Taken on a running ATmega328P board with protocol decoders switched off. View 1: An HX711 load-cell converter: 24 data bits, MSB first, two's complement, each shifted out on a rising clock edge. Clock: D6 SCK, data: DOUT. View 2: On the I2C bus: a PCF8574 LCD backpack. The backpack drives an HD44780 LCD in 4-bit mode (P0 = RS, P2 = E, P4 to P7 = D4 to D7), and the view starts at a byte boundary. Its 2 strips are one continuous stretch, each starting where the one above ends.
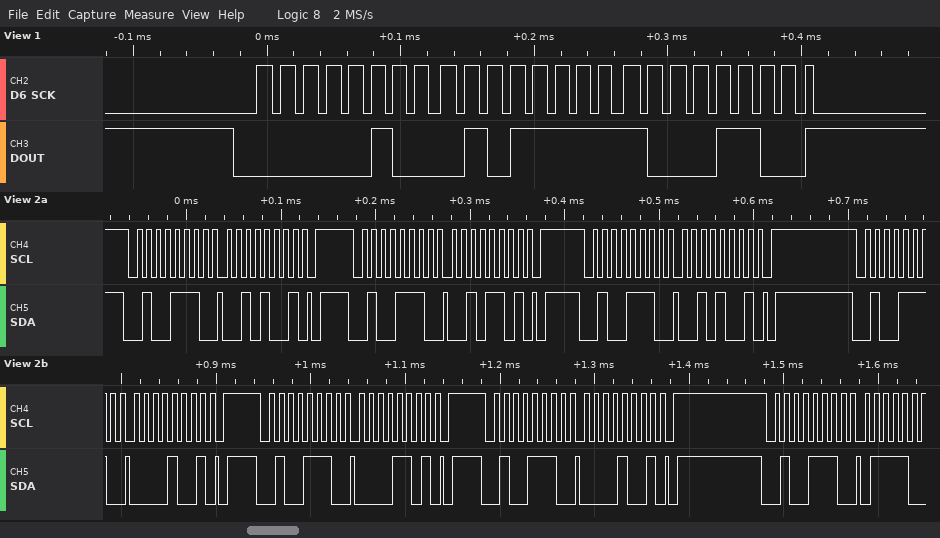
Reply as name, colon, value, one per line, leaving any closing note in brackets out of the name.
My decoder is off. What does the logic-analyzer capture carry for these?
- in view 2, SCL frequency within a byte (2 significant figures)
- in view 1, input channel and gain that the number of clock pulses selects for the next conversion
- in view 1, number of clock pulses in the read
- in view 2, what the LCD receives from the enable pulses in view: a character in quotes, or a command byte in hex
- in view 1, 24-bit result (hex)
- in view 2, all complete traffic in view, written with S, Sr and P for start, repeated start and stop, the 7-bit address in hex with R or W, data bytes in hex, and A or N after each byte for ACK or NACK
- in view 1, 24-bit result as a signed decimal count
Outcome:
in view 2, SCL frequency within a byte: 100 kHz
in view 1, input channel and gain that the number of clock pulses selects for the next conversion: channel A, gain 128
in view 1, number of clock pulses in the read: 25
in view 2, what the LCD receives from the enable pulses in view: a character in quotes, or a command byte in hex: ' '
in view 1, 24-bit result: 0x045F8C
in view 2, all complete traffic in view, written with S, Sr and P for start, repeated start and stop, the 7-bit address in hex with R or W, data bytes in hex, and A or N after each byte for ACK or NACK: S 27W A 29 A P S 27W A 2D A P S 27W A 29 A P S 27W A 09 A P S 27W A 0D A P S 27W A 09 A P S 27W A
in view 1, 24-bit result as a signed decimal count: 286604
